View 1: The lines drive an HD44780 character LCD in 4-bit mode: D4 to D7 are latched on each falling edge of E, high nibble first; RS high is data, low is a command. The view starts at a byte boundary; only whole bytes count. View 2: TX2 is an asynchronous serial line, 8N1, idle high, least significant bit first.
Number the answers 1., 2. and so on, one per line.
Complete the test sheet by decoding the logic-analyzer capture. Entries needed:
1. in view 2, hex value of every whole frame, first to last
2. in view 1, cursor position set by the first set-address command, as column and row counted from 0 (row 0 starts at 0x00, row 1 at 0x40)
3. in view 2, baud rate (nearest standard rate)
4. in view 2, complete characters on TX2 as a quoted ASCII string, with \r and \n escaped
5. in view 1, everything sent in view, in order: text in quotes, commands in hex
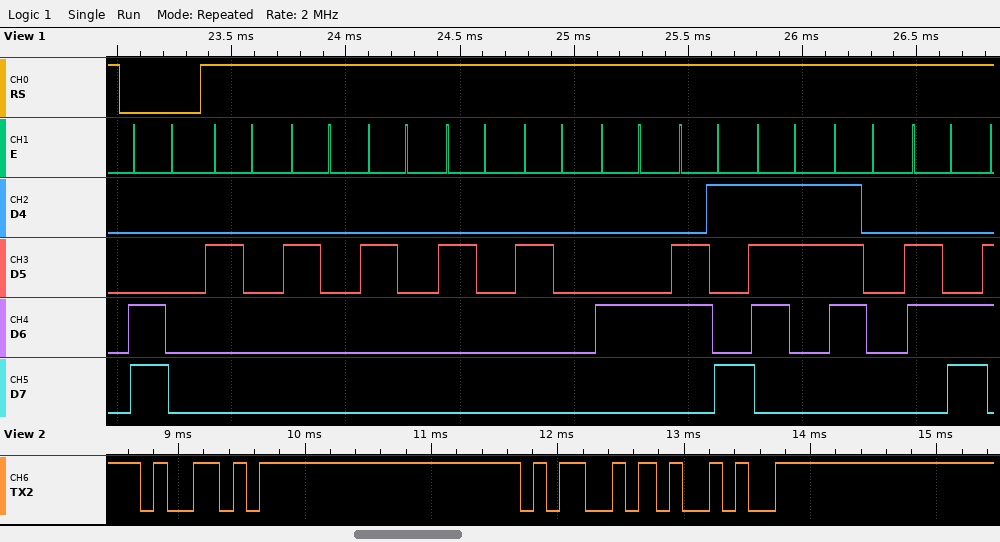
1. 59 4D 29
2. column 0, row 1
3. 9600 baud
4. "YM)"
5. 0xC0 "     Displ"
